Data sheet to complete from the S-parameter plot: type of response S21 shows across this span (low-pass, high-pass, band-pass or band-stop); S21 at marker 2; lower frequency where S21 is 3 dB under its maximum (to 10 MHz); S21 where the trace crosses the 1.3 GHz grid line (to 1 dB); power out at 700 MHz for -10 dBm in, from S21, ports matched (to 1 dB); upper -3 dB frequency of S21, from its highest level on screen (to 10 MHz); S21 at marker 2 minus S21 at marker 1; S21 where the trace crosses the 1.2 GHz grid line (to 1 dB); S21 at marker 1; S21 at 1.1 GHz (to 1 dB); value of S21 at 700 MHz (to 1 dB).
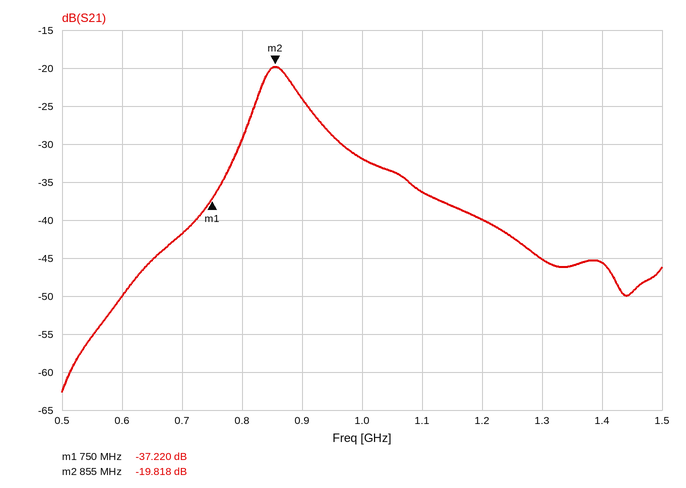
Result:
band-pass
-19.818 dB
830 MHz
-45 dB
-52 dBm
890 MHz
17.402 dB
-40 dB
-37.220 dB
-36 dB
-42 dB
